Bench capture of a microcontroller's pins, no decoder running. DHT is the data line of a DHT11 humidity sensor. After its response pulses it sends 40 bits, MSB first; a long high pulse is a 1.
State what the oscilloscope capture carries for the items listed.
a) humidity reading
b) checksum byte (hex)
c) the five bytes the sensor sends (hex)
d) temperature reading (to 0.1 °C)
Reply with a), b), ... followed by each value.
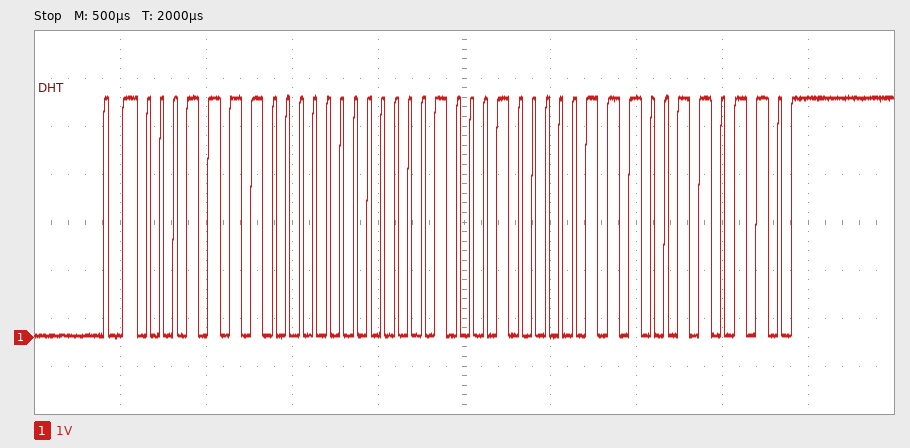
a) 30 %
b) 0x36
c) 1E 00 11 07 36
d) 17.7 °C
